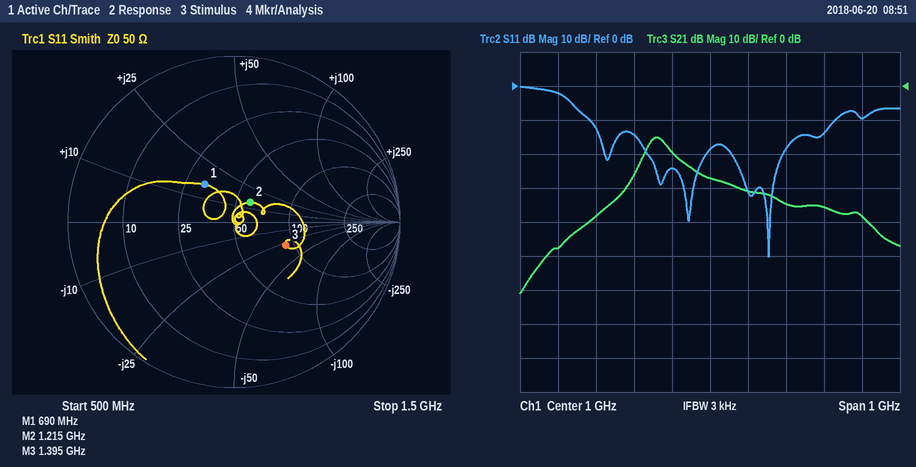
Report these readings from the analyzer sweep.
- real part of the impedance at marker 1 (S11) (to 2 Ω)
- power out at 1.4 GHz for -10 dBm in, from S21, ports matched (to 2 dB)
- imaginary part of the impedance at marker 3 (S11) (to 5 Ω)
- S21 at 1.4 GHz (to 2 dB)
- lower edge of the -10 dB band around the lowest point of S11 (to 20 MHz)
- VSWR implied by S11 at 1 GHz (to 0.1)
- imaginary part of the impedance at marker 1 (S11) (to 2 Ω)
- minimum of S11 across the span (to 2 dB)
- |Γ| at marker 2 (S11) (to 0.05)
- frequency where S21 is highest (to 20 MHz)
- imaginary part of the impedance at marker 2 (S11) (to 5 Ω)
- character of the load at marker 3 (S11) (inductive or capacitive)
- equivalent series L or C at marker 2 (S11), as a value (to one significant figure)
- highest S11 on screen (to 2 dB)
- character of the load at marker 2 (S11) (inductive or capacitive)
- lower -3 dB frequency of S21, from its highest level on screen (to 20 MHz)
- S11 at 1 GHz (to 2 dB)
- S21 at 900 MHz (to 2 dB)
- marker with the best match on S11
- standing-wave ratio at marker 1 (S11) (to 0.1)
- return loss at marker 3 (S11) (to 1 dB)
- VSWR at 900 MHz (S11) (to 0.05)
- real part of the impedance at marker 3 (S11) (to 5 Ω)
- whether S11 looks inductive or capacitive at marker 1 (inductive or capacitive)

32 Ω
-48 dBm
-30 Ω
-38 dB
680 MHz
1.3
+16 Ω
-50 dB
0.15
860 MHz
+15 Ω
capacitive
2 nH
0 dB
inductive
840 MHz
-18 dB
-20 dB
marker 2
1.8
9 dB
1.15
90 Ω
inductive
